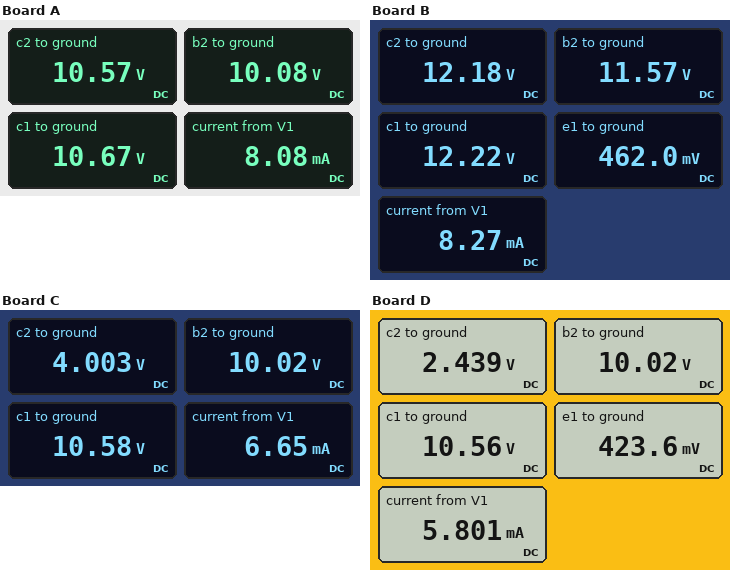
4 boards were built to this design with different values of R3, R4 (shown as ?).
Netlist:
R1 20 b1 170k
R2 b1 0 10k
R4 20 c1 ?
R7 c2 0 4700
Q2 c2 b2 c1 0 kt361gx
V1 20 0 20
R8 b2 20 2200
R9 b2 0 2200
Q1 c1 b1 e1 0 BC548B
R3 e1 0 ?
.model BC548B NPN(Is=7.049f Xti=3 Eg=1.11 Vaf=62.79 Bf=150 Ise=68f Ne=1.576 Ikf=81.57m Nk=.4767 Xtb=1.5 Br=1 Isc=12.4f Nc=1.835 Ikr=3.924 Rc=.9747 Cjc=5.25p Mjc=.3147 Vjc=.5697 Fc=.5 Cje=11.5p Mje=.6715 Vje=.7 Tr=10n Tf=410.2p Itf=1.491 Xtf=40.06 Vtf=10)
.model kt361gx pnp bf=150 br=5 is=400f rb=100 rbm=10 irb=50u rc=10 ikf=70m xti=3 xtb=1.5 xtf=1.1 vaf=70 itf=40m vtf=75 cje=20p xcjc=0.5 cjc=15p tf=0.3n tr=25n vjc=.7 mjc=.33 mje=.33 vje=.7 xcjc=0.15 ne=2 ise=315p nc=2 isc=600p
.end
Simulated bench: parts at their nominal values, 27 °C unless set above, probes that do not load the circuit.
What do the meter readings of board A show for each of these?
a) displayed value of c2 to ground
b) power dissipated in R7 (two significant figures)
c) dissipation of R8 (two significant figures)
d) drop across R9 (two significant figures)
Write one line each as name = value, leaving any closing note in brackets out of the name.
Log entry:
displayed value of c2 to ground = 10.57 V
power dissipated in R7 = 24 mW
dissipation of R8 = 45 mW
drop across R9 = 10 V
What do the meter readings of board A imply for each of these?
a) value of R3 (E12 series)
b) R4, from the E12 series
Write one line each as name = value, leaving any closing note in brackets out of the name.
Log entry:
value of R3 = 330 Ω
R4, from the E12 series = 2.7 kΩ
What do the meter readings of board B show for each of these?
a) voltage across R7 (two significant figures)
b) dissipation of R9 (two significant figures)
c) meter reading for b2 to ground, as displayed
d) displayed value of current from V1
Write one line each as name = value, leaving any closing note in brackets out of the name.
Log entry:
voltage across R7 = 12 V
dissipation of R9 = 61 mW
meter reading for b2 to ground, as displayed = 11.57 V
displayed value of current from V1 = 8.27 mA
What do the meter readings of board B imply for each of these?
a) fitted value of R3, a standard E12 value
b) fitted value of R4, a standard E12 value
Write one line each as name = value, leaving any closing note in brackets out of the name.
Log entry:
fitted value of R3, a standard E12 value = 1.5 kΩ
fitted value of R4, a standard E12 value = 1.8 kΩ
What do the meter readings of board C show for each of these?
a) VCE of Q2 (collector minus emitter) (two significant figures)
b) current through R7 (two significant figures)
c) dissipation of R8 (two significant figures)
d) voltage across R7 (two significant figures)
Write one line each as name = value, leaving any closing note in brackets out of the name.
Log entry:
VCE of Q2 (collector minus emitter) = -6.6 V
current through R7 = 850 µA
dissipation of R8 = 45 mW
voltage across R7 = 4.0 V
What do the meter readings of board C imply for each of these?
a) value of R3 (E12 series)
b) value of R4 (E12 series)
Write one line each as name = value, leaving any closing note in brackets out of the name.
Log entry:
value of R3 = 330 Ω
value of R4 = 4.7 kΩ
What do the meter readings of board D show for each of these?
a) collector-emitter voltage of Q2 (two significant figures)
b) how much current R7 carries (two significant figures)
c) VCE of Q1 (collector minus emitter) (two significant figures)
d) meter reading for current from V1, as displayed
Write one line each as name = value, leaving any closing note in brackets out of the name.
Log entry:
collector-emitter voltage of Q2 = -8.1 V
how much current R7 carries = 520 µA
VCE of Q1 (collector minus emitter) = 10 V
meter reading for current from V1, as displayed = 5.801 mA
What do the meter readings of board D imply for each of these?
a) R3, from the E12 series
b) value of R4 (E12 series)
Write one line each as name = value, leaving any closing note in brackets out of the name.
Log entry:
R3, from the E12 series = 680 Ω
value of R4 = 8.2 kΩ
